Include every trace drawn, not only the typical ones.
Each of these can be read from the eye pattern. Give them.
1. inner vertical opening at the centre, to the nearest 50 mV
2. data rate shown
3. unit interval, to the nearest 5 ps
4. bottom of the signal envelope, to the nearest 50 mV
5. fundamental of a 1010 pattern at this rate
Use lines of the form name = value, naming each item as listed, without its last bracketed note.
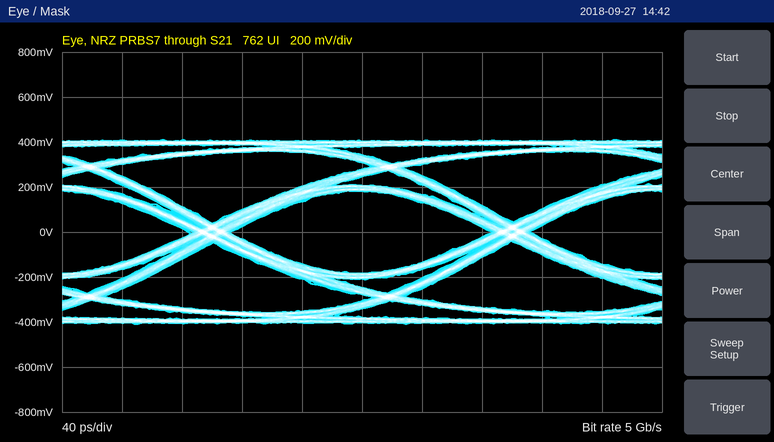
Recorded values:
inner vertical opening at the centre, to the nearest 50 mV = 350 mV
data rate shown = 5 Gb/s
unit interval, to the nearest 5 ps = 200 ps
bottom of the signal envelope, to the nearest 50 mV = -400 mV
fundamental of a 1010 pattern at this rate = 2.5 GHz
